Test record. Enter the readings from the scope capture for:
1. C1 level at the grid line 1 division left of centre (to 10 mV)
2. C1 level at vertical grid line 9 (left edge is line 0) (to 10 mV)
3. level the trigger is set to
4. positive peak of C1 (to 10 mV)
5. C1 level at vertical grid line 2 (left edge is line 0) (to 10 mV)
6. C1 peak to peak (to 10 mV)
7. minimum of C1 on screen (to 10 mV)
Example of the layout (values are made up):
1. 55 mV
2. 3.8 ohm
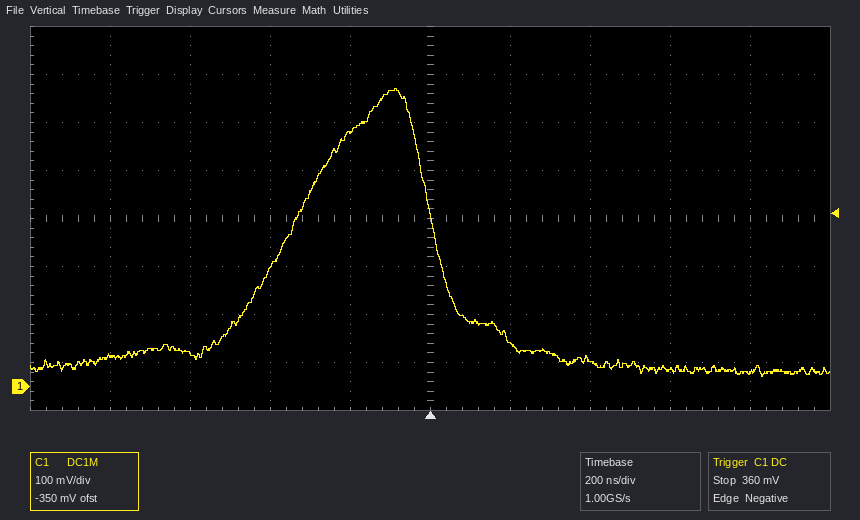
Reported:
1. 530 mV
2. 30 mV
3. 360 mV
4. 620 mV
5. 70 mV
6. 600 mV
7. 20 mV
